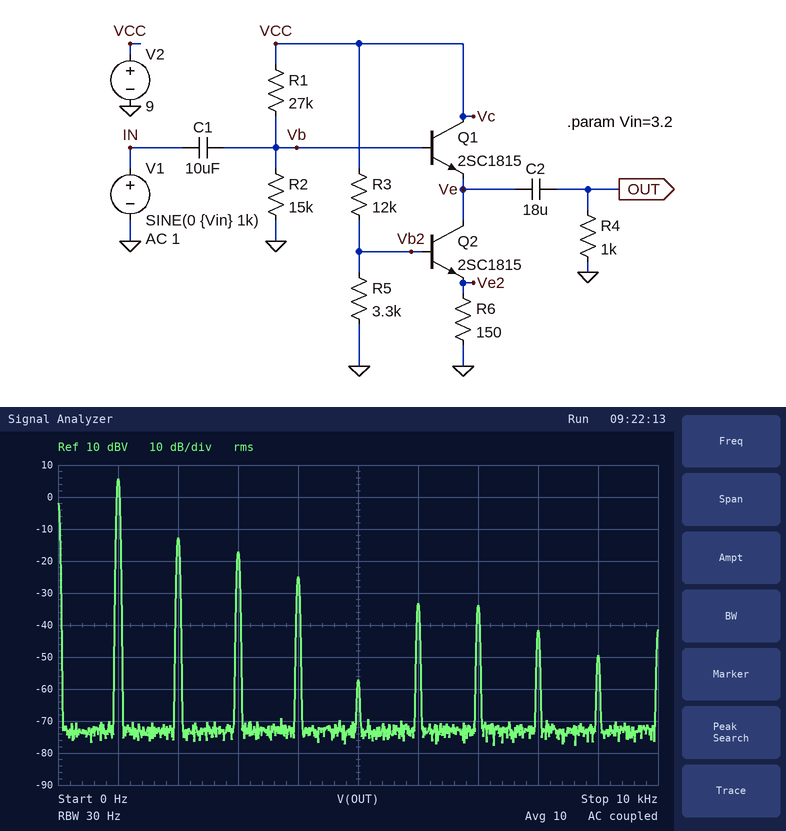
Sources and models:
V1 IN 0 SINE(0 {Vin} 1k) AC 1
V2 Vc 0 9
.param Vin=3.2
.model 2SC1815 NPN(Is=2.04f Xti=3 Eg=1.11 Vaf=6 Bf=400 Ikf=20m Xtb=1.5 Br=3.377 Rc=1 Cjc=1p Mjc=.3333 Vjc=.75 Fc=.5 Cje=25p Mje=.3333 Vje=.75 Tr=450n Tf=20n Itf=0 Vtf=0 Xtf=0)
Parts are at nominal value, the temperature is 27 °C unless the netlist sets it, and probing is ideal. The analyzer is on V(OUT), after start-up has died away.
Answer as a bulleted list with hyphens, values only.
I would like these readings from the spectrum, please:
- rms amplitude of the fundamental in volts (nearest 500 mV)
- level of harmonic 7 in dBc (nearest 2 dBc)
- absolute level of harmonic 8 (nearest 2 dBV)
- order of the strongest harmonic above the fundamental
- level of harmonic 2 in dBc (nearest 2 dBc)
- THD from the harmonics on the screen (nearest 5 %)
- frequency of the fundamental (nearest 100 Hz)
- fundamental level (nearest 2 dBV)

- 2.0 V
- -40 dBc
- -42 dBV
- 2
- -18 dBc
- 15 %
- 1.0 kHz
- 6 dBV
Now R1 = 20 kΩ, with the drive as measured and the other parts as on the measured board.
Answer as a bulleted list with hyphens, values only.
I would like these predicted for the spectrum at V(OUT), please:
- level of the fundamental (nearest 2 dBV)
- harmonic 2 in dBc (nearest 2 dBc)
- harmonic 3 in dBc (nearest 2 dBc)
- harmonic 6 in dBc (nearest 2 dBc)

- 6 dBV
- -26 dBc
- -28 dBc
- -44 dBc
